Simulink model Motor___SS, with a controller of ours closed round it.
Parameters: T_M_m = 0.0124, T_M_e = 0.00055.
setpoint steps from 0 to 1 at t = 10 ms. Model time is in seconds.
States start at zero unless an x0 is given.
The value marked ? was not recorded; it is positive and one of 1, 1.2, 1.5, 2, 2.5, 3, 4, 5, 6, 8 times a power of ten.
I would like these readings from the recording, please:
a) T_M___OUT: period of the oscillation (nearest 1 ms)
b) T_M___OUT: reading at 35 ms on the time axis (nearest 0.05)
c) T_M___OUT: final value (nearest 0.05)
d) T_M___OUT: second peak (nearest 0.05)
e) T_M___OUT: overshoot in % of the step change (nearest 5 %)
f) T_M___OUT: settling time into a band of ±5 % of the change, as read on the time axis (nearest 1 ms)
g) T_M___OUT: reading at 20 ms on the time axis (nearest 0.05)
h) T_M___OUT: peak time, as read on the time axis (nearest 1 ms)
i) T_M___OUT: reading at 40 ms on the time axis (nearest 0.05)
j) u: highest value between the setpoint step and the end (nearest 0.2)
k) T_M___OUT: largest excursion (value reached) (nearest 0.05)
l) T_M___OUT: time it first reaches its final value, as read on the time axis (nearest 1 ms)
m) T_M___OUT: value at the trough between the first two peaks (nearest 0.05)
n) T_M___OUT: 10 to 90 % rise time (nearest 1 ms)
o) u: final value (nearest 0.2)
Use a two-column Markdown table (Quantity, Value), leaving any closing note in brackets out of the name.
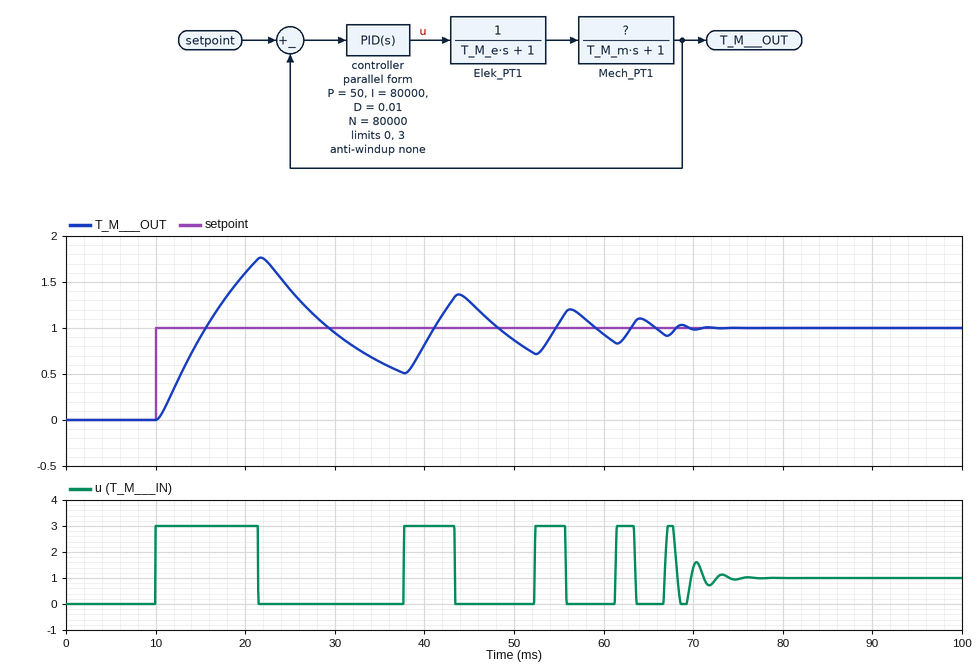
| Quantity | Value |
|---|---|
| T_M___OUT: period of the oscillation | 22 ms |
| T_M___OUT: reading at 35 ms on the time axis | 0.65 |
| T_M___OUT: final value | 1.00 |
| T_M___OUT: second peak | 1.35 |
| T_M___OUT: overshoot in % of the step change | 75 % |
| T_M___OUT: settling time into a band of ±5 % of the change, as read on the time axis | 68 ms |
| T_M___OUT: reading at 20 ms on the time axis | 1.60 |
| T_M___OUT: peak time, as read on the time axis | 22 ms |
| T_M___OUT: reading at 40 ms on the time axis | 0.80 |
| u: highest value between the setpoint step and the end | 3.0 |
| T_M___OUT: largest excursion (value reached) | 1.75 |
| T_M___OUT: time it first reaches its final value, as read on the time axis | 16 ms |
| T_M___OUT: value at the trough between the first two peaks | 0.50 |
| T_M___OUT: 10 to 90 % rise time | 4 ms |
| u: final value | 1.0 |
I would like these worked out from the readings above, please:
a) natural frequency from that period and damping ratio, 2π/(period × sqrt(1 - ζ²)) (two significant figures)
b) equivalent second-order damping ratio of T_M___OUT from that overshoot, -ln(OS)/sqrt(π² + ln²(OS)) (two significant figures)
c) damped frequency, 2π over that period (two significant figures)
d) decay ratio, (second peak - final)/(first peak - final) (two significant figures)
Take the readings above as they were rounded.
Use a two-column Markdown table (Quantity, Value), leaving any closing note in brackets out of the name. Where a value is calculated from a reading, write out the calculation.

| Quantity | Value |
|---|---|
| natural frequency from that period and damping ratio, 2π/(period × sqrt(1 - ζ²)) | 2π / (22 × sqrt(1 - 0.091²)) = 0.29 rad/ms |
| equivalent second-order damping ratio of T_M___OUT from that overshoot, -ln(OS)/sqrt(π² + ln²(OS)) | ln(0.75) = -0.288; 0.288 / sqrt(9.870 + 0.083) = 0.091 |
| damped frequency, 2π over that period | 2π / 22 = 0.29 rad/ms |
| decay ratio, (second peak - final)/(first peak - final) | (1.35 - 1) / (1.75 - 1) = 0.47 |
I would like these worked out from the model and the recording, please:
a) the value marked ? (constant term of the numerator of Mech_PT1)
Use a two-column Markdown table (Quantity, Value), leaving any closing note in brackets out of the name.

| Quantity | Value |
|---|---|
| the value marked ? | 1 |
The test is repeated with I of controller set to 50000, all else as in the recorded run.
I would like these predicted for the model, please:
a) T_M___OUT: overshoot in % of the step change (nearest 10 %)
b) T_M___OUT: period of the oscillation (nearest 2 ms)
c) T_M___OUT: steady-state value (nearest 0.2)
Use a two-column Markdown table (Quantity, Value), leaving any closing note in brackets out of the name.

| Quantity | Value |
|---|---|
| T_M___OUT: overshoot in % of the step change | 70 % |
| T_M___OUT: period of the oscillation | 20 ms |
| T_M___OUT: steady-state value | 1.0 |
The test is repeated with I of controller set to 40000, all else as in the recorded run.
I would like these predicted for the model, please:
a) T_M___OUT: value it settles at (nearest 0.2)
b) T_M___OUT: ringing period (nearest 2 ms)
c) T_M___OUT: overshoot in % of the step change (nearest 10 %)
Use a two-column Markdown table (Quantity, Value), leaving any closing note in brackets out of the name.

| Quantity | Value |
|---|---|
| T_M___OUT: value it settles at | 1.0 |
| T_M___OUT: ringing period | 18 ms |
| T_M___OUT: overshoot in % of the step change | 70 % |
